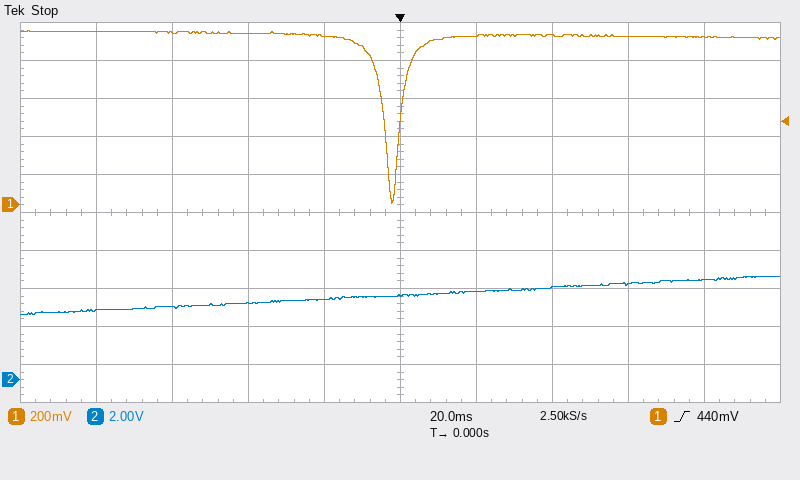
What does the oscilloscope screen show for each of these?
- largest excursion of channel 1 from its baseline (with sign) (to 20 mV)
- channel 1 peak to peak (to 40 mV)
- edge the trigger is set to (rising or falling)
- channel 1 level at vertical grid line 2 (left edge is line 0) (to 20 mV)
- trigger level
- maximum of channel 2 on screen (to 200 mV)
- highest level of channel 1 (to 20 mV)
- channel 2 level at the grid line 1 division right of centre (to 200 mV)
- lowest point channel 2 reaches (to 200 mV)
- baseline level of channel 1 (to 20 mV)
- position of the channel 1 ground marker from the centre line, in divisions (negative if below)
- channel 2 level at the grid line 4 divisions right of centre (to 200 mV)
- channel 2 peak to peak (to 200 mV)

-880 mV
920 mV
rising
900 mV
440 mV
5.4 V
920 mV
4.6 V
3.4 V
900 mV
+0.2 div
5.2 V
2.0 V
